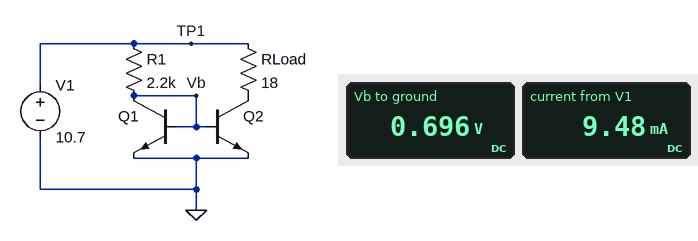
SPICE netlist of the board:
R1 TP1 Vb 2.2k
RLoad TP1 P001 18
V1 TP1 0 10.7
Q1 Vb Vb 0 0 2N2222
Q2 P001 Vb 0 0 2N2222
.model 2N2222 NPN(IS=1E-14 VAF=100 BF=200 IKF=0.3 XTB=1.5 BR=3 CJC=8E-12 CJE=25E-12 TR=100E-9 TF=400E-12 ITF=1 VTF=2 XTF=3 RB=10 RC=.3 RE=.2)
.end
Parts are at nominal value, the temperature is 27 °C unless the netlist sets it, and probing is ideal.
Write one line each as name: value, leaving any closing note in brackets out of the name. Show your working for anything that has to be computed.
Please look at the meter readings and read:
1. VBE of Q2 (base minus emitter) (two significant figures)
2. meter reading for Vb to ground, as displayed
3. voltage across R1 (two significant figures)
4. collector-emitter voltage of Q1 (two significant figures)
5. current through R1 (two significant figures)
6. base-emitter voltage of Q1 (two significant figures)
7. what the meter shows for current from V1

VBE of Q2 (base minus emitter): 696 mV = 700 mV
meter reading for Vb to ground, as displayed: 0.696 V
voltage across R1: 10.7 V - 696 mV = 10 V
collector-emitter voltage of Q1: 696 mV = 700 mV
current through R1: (10.7 V - 696 mV) / 2.2 kΩ = 4.5 mA
base-emitter voltage of Q1: 696 mV = 700 mV
what the meter shows for current from V1: 9.48 mA
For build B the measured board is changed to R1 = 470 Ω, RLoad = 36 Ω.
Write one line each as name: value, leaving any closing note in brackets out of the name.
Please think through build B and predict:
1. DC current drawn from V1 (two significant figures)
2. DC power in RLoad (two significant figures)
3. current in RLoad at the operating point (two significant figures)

DC current drawn from V1: 44 mA
DC power in RLoad: 18 mW
current in RLoad at the operating point: 23 mA
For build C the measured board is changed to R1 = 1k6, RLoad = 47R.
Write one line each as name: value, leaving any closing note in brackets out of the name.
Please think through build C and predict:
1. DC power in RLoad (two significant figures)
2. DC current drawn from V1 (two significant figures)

DC power in RLoad: 2.1 mW
DC current drawn from V1: 13 mA
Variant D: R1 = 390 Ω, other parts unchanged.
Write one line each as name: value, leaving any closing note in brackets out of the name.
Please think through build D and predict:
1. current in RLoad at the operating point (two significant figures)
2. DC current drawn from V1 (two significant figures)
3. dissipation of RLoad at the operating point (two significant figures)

current in RLoad at the operating point: 27 mA
DC current drawn from V1: 53 mA
dissipation of RLoad at the operating point: 13 mW
